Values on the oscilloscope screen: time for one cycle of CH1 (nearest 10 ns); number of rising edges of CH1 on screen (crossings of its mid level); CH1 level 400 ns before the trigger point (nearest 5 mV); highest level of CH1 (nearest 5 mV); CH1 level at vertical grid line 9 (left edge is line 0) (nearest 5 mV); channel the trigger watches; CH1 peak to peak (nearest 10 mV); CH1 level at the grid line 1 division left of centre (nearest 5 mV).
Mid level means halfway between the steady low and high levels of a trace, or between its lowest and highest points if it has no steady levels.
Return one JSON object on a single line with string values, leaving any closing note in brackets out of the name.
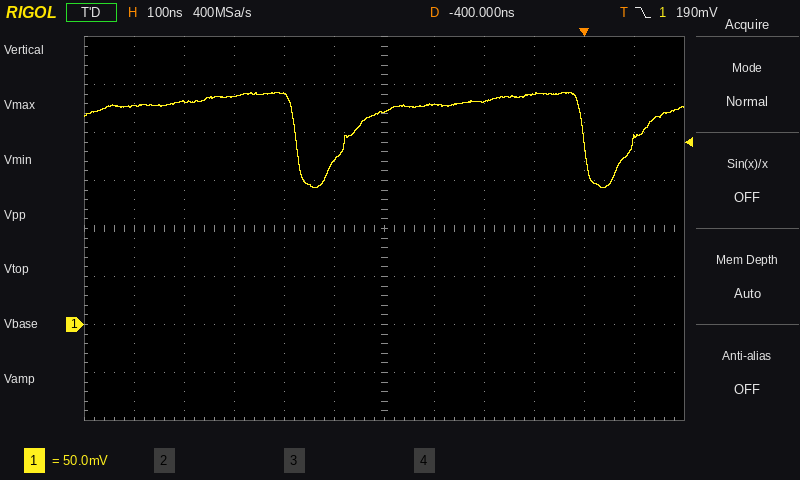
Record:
{"time for one cycle of CH1": "580 ns", "number of rising edges of CH1 on screen": "2", "CH1 level 400 ns before the trigger point": "220 mV", "highest level of CH1": "240 mV", "CH1 level at vertical grid line 9 (left edge is line 0)": "240 mV", "channel the trigger watches": "CH1", "CH1 peak to peak": "100 mV", "CH1 level at the grid line 1 division left of centre": "170 mV"}
